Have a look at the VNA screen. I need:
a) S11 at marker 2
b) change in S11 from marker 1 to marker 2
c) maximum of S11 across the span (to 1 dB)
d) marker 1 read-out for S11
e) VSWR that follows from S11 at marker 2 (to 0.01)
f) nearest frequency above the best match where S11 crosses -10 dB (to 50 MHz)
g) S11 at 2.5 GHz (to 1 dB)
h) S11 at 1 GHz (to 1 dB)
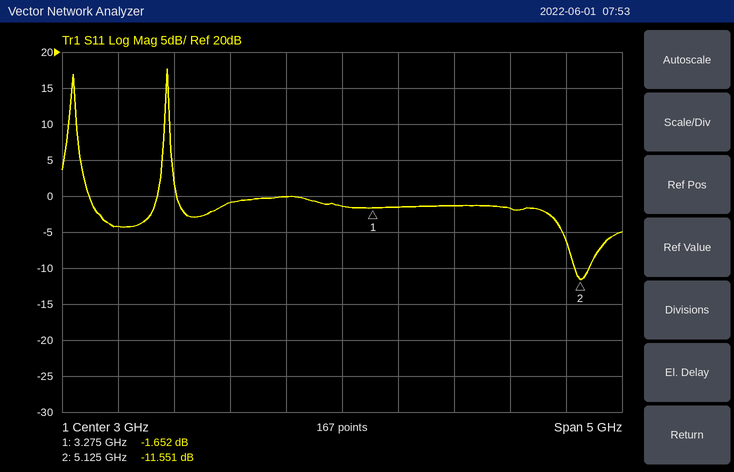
-11.551 dB
-9.899 dB
18 dB
-1.652 dB
1.72
5.20 GHz
0 dB
-4 dB
